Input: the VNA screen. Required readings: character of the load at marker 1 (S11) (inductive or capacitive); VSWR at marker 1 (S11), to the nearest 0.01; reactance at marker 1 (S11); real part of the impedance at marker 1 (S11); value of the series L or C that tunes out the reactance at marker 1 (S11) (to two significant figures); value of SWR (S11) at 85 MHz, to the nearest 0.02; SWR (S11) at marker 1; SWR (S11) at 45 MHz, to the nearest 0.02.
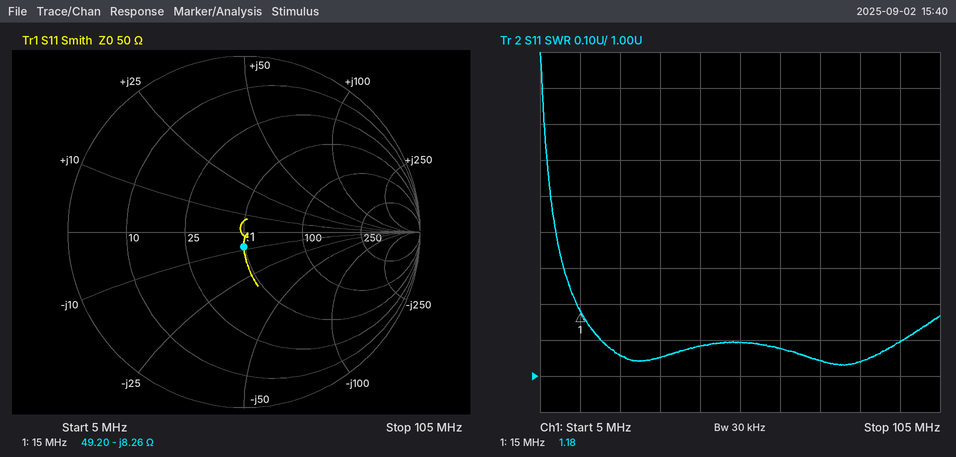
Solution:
capacitive
1.18
-8.26 Ω
49.20 Ω
88 nH
1.04
1.18
1.08
